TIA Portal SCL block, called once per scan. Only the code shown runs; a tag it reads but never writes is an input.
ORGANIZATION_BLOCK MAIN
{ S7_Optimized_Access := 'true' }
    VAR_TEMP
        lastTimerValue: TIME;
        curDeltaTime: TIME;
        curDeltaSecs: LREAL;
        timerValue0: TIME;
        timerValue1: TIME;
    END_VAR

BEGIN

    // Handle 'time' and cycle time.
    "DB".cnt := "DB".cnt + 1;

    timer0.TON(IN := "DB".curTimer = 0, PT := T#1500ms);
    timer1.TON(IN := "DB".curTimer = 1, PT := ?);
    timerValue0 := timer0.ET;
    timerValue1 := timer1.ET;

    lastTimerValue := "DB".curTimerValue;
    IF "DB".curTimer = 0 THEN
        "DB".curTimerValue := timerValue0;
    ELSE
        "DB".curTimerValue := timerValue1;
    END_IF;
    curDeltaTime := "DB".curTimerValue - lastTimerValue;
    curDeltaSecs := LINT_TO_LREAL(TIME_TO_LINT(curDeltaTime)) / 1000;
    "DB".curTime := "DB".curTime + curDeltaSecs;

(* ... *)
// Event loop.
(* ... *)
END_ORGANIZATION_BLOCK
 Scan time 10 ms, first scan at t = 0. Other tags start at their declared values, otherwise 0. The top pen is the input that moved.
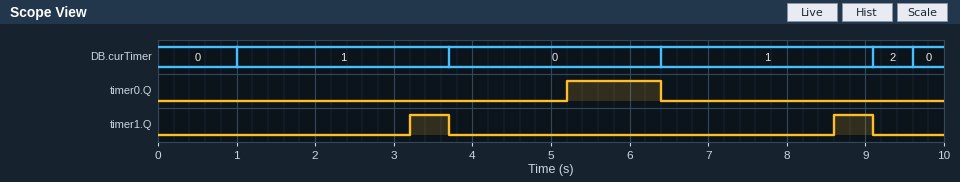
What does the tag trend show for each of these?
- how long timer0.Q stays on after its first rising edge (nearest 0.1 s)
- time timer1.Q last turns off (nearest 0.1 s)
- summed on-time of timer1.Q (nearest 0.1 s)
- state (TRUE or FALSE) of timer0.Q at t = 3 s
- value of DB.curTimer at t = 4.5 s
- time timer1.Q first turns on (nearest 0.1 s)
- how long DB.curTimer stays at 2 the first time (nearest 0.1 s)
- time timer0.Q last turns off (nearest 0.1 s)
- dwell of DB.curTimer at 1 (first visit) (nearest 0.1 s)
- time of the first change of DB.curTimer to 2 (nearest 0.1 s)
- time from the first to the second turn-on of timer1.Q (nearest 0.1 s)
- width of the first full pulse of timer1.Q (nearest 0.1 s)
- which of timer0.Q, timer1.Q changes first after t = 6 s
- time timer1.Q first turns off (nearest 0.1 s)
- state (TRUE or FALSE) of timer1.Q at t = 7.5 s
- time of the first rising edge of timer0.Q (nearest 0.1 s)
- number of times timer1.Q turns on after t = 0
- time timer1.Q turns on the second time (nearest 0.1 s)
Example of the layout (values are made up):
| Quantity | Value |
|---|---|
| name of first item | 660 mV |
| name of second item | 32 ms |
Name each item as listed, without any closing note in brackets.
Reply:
| Quantity | Value |
|---|---|
| how long timer0.Q stays on after its first rising edge | 1.2 s |
| time timer1.Q last turns off | 9.1 s |
| summed on-time of timer1.Q | 1.0 s |
| state (TRUE or FALSE) of timer0.Q at t = 3 s | FALSE |
| value of DB.curTimer at t = 4.5 s | 0 |
| time timer1.Q first turns on | 3.2 s |
| how long DB.curTimer stays at 2 the first time | 0.5 s |
| time timer0.Q last turns off | 6.4 s |
| dwell of DB.curTimer at 1 (first visit) | 2.7 s |
| time of the first change of DB.curTimer to 2 | 9.1 s |
| time from the first to the second turn-on of timer1.Q | 5.4 s |
| width of the first full pulse of timer1.Q | 0.5 s |
| which of timer0.Q, timer1.Q changes first after t = 6 s | timer0.Q |
| time timer1.Q first turns off | 3.7 s |
| state (TRUE or FALSE) of timer1.Q at t = 7.5 s | FALSE |
| time of the first rising edge of timer0.Q | 5.2 s |
| number of times timer1.Q turns on after t = 0 | 2 |
| time timer1.Q turns on the second time | 8.6 s |
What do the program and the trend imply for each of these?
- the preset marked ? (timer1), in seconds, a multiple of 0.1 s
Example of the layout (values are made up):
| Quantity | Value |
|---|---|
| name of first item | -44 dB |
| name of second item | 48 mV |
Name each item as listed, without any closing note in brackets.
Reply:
| Quantity | Value |
|---|---|
| the preset marked ? (timer1), in seconds, a multiple of 0.1 s | 2.2 s |
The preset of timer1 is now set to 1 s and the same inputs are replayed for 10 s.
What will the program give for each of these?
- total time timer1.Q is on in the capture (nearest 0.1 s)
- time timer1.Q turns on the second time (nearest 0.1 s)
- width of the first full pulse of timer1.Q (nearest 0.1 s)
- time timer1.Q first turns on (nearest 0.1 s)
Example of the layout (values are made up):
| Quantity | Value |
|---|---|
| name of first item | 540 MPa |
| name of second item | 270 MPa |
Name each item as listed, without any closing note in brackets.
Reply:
| Quantity | Value |
|---|---|
| total time timer1.Q is on in the capture | 3.4 s |
| time timer1.Q turns on the second time | 7.4 s |
| width of the first full pulse of timer1.Q | 1.7 s |
| time timer1.Q first turns on | 2.0 s |
